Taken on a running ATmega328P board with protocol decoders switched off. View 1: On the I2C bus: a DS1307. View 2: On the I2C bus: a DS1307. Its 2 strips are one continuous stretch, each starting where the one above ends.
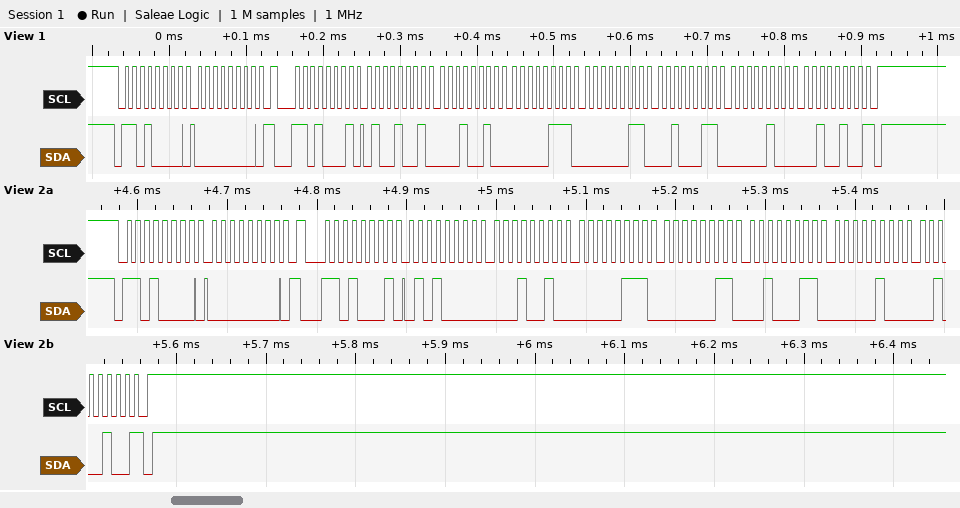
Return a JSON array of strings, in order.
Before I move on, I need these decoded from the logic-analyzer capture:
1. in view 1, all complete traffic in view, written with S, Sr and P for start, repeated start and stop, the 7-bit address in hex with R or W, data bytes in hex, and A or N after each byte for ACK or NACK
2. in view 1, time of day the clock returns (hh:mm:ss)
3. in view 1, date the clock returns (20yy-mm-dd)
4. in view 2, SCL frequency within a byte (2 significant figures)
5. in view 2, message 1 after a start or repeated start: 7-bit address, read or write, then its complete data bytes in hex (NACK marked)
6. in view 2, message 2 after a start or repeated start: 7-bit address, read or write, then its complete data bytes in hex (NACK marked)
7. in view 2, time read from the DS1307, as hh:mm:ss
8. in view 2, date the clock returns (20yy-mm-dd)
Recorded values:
["S 68W A 00 A Sr 68R A 49 A 12 A 07 A 03 A 23 A 04 A 24 N P", "07:12:49", "2024-04-23", "100 kHz", "0x68 write: 00", "0x68 read: 50 12 07 03 23 04 24 NACK", "07:12:50", "2024-04-23"]
